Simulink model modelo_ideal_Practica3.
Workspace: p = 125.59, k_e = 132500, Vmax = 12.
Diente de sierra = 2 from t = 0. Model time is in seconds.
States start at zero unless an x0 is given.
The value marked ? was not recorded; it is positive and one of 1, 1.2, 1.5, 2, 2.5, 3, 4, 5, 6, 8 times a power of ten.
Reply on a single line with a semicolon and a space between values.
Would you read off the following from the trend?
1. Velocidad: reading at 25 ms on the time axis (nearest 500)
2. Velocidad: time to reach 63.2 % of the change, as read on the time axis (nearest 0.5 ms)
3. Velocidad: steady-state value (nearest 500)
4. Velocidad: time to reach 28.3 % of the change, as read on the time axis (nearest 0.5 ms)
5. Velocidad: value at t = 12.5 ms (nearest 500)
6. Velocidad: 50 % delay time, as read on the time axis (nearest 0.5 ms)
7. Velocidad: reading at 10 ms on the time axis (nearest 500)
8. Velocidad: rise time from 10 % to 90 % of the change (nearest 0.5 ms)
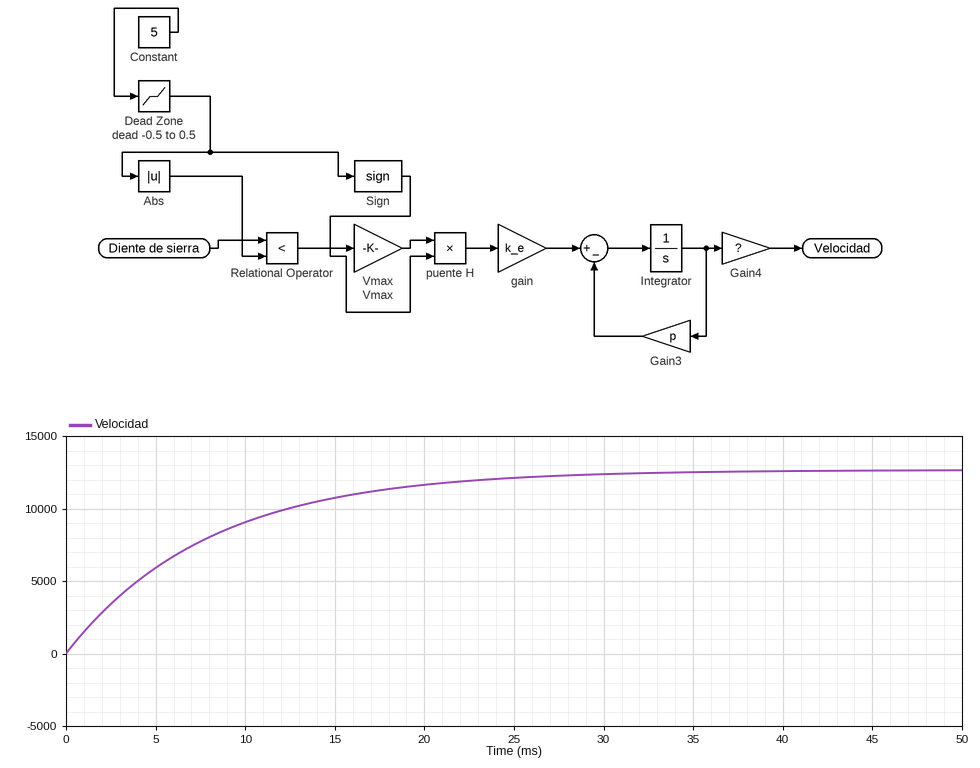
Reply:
12000; 8.0 ms; 12500; 2.5 ms; 10000; 5.5 ms; 9000; 17.5 ms
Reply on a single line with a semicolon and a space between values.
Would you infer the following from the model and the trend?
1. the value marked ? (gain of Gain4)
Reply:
1
